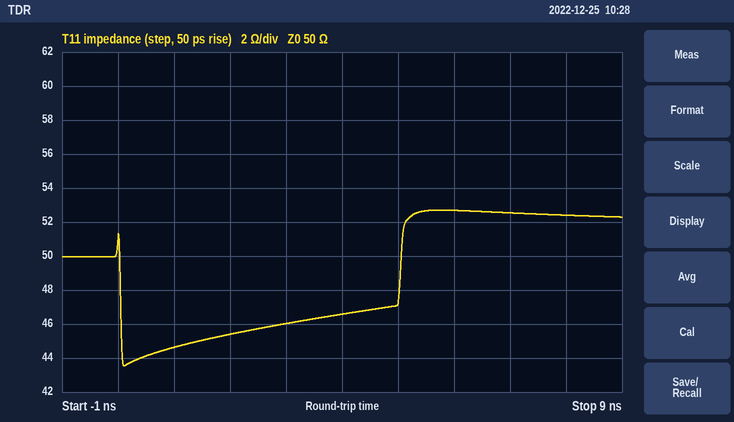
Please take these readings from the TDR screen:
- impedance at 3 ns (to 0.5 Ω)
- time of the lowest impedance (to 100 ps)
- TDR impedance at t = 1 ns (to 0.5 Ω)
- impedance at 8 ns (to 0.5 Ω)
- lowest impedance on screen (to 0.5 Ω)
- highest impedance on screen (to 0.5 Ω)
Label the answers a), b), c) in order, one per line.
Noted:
a) 46.0 Ω
b) 100 ps
c) 44.5 Ω
d) 52.5 Ω
e) 43.5 Ω
f) 52.5 Ω
